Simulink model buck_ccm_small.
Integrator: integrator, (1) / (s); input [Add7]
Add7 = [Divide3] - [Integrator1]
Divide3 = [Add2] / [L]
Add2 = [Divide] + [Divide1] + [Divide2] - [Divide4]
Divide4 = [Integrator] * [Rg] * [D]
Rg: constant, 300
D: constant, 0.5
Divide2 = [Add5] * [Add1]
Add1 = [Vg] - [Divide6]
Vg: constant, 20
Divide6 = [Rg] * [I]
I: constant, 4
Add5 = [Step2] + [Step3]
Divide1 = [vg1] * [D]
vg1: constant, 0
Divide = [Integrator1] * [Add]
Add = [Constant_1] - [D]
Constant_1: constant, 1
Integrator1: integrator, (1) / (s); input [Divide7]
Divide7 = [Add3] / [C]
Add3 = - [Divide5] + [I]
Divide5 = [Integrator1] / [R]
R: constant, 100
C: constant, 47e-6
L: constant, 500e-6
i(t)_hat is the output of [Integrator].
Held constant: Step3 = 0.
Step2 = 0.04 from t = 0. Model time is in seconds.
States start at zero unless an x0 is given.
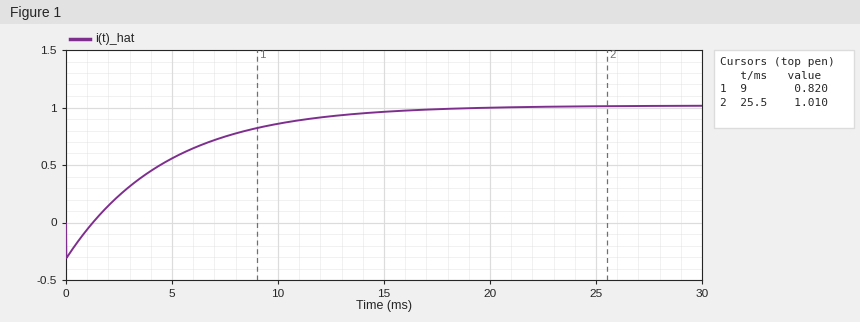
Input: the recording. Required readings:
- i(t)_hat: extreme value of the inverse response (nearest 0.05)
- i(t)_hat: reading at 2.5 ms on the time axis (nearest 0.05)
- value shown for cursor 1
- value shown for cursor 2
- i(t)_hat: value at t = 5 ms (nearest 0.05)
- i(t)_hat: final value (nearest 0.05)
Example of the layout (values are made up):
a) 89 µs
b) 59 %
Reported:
a) -0.30
b) 0.25
c) 0.820
d) 1.010
e) 0.55
f) 1.00
